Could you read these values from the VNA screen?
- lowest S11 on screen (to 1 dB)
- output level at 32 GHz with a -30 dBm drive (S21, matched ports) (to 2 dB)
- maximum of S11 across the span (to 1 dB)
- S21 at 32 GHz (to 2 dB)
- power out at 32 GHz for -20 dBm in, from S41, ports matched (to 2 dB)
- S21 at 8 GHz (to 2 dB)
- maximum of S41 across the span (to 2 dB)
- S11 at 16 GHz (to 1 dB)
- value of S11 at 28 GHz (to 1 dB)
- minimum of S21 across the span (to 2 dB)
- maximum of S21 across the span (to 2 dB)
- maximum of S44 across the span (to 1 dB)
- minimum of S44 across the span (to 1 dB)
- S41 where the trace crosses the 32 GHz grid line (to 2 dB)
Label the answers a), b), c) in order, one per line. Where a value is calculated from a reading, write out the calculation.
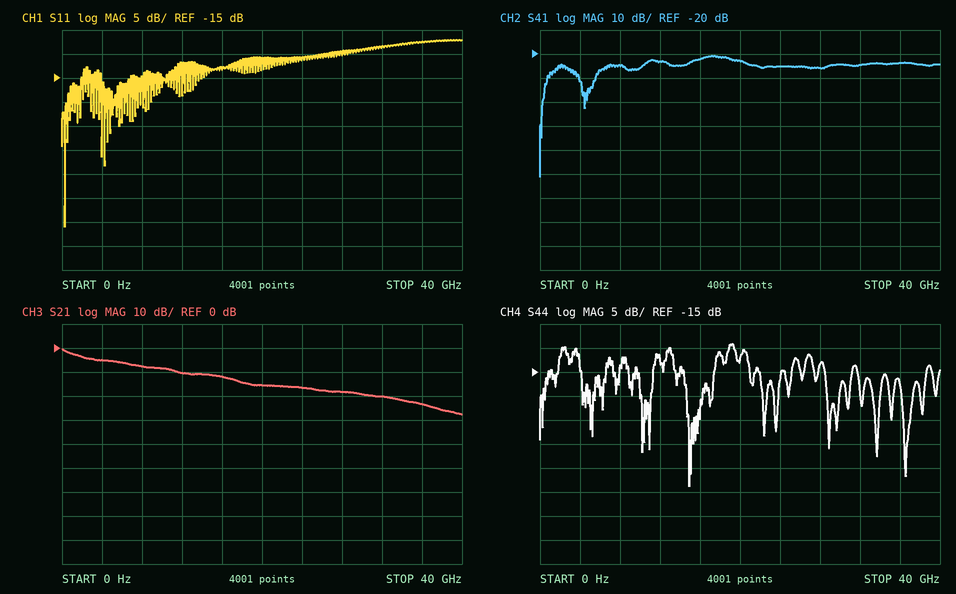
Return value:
a) -46 dB
b) -30 dBm + (-20 dB) = -50 dBm
c) -7 dB
d) -20 dB
e) -20 dBm + (-24 dB) = -44 dBm
f) -8 dB
g) -20 dB
h) -13 dB
i) -10 dB
j) -28 dB
k) 0 dB
l) -9 dB
m) -39 dB
n) -24 dB
